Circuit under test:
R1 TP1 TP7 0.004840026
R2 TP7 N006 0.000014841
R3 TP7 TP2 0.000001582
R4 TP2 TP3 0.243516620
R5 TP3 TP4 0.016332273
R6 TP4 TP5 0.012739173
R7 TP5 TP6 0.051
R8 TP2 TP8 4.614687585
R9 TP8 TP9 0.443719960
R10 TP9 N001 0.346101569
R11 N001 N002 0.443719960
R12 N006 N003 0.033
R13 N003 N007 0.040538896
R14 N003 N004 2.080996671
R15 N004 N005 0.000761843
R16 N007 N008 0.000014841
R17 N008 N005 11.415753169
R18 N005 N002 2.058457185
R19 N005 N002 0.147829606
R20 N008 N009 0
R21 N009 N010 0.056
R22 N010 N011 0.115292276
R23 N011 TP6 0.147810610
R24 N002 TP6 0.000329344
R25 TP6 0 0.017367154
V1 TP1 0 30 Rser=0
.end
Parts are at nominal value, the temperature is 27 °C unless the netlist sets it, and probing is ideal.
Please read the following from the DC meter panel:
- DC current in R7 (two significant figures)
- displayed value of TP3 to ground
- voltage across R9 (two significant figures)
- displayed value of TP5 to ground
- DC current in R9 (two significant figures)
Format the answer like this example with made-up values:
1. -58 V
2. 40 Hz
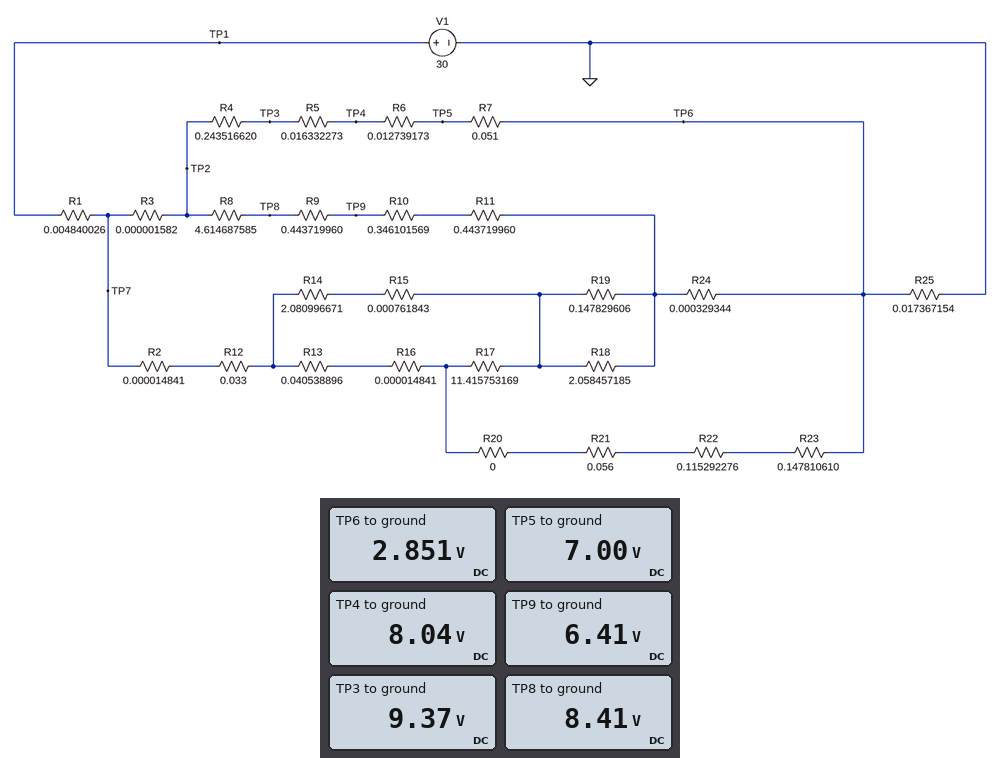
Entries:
1. 81 A
2. 9.37 V
3. 2.0 V
4. 7.00 V
5. 4.5 A
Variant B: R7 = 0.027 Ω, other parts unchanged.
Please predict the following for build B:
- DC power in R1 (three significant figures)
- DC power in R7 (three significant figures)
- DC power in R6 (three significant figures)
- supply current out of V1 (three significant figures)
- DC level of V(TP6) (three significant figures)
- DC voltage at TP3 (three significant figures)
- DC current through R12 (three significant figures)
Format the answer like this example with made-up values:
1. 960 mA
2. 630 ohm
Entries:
1. 140 W
2. 207 W
3. 97.6 W
4. 170 A
5. 2.95 V
6. 7.86 V
7. 77.8 A
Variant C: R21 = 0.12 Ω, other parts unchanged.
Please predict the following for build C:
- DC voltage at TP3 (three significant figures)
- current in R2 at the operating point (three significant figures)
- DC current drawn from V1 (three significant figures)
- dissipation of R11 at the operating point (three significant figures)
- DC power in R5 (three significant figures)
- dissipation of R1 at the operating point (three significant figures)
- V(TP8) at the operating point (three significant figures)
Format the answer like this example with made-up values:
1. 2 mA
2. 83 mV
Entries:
1. 9.28 V
2. 69.6 A
3. 156 A
4. 9.13 W
5. 110 W
6. 118 W
7. 8.31 V
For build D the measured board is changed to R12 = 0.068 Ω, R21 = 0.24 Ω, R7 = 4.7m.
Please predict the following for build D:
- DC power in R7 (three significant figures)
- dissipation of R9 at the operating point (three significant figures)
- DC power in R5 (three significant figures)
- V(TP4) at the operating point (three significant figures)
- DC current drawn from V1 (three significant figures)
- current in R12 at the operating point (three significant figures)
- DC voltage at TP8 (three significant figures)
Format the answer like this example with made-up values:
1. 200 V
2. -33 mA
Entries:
1. 43.2 W
2. 9.16 W
3. 150 W
4. 4.35 V
5. 154 A
6. 53.9 A
7. 8.29 V
